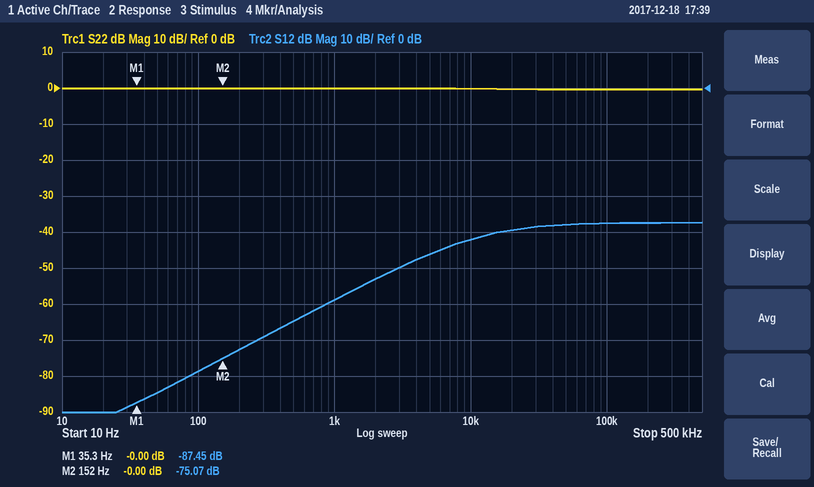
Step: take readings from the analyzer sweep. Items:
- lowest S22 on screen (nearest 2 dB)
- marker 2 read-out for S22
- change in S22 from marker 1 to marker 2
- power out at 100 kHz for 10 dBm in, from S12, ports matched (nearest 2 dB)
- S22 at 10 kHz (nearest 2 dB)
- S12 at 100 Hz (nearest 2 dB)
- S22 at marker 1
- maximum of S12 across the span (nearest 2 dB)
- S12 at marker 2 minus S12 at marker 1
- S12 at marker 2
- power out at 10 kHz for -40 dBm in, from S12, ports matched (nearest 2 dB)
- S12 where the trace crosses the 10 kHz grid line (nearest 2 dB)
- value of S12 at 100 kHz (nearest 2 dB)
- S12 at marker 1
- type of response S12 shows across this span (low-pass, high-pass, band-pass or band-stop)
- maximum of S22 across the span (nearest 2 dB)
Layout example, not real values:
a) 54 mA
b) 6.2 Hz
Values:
a) 0 dB
b) -0.00 dB
c) 0.00 dB
d) -28 dBm
e) 0 dB
f) -78 dB
g) -0.00 dB
h) -38 dB
i) 12.38 dB
j) -75.07 dB
k) -82 dBm
l) -42 dB
m) -38 dB
n) -87.45 dB
o) high-pass
p) 0 dB
